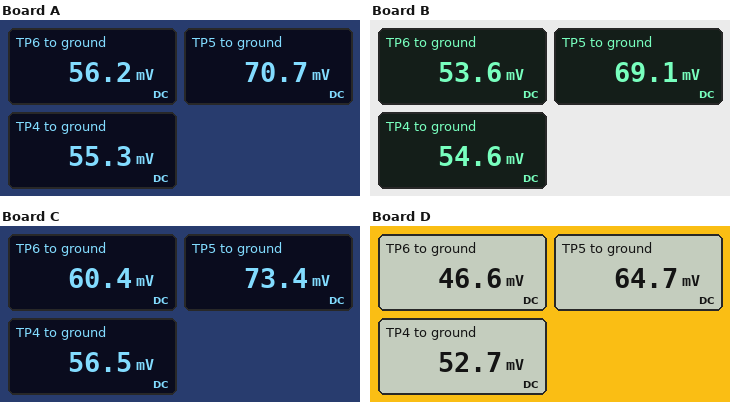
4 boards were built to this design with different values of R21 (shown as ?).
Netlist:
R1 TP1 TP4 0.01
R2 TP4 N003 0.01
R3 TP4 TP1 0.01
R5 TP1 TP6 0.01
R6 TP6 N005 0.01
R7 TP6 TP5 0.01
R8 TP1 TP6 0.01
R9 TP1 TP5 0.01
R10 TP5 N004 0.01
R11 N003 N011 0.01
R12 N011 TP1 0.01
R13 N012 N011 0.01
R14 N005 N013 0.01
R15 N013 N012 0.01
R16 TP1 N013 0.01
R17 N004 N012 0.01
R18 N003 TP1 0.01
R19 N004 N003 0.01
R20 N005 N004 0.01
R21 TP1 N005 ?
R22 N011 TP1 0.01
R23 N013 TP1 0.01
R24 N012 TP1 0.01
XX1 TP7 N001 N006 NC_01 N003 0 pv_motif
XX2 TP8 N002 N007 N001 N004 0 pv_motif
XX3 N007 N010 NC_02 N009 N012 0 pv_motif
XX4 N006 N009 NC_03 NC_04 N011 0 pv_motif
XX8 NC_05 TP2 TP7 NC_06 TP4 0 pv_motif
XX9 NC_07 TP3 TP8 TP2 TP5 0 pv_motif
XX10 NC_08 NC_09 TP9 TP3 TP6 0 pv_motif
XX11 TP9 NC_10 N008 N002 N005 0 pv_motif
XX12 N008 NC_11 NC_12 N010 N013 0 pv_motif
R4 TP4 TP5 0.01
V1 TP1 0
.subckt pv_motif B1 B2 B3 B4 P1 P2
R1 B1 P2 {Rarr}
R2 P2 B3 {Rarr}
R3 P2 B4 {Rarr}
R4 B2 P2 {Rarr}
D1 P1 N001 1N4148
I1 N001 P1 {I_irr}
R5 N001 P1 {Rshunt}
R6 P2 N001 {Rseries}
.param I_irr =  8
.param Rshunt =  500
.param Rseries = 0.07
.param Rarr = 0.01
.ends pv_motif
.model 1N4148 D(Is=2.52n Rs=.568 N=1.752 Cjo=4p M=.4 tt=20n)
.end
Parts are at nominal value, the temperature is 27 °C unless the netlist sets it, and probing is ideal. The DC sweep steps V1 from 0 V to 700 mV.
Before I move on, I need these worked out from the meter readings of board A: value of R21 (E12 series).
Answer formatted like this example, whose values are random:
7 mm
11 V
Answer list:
0.012 Ω
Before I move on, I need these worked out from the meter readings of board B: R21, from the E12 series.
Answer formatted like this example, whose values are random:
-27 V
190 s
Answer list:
8.2 mΩ
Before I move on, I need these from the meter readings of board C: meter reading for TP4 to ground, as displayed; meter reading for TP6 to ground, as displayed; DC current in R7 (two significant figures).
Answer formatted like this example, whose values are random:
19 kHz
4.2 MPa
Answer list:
56.5 mV
60.4 mV
1.3 A
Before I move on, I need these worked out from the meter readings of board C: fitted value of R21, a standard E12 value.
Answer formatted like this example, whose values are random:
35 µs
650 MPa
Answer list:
0.027 Ω
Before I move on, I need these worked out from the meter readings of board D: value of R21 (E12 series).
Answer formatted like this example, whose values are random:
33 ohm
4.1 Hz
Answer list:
3.3 mΩ
